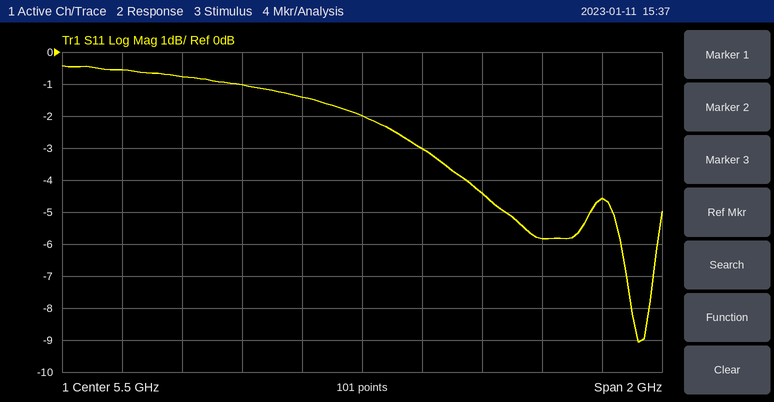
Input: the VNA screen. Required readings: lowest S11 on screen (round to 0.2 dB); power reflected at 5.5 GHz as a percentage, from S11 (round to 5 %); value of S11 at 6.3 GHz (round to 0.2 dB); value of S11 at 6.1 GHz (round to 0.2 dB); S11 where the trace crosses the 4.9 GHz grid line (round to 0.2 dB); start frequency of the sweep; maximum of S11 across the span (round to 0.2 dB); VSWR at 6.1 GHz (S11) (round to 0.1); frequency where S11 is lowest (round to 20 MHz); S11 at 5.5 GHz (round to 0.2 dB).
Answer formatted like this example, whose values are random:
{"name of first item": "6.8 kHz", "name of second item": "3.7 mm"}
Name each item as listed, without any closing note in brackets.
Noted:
{"lowest S11 on screen": "-9.0 dB", "power reflected at 5.5 GHz as a percentage, from S11": "65 %", "value of S11 at 6.3 GHz": "-4.6 dB", "value of S11 at 6.1 GHz": "-5.8 dB", "S11 where the trace crosses the 4.9 GHz grid line": "-0.8 dB", "start frequency of the sweep": "4.5 GHz", "maximum of S11 across the span": "-0.4 dB", "VSWR at 6.1 GHz (S11)": "3.1", "frequency where S11 is lowest": "6.42 GHz", "S11 at 5.5 GHz": "-2.0 dB"}
